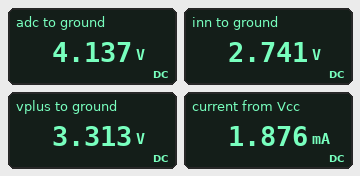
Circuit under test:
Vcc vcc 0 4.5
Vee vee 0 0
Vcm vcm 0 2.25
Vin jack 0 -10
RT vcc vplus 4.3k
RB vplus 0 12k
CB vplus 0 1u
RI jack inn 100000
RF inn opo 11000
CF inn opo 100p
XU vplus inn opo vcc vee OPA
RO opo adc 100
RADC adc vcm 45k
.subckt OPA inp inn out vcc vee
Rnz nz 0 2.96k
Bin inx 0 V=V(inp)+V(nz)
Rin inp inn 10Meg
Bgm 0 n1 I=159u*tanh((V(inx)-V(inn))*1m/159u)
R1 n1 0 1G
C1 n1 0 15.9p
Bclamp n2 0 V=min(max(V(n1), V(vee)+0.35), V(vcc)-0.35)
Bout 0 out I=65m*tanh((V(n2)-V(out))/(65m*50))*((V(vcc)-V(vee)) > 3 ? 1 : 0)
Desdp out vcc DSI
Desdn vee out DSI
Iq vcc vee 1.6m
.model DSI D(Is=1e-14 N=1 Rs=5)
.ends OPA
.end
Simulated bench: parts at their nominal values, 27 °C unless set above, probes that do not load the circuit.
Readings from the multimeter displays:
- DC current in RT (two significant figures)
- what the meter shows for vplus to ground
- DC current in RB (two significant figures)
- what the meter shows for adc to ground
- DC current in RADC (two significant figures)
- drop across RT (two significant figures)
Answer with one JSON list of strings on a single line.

["280 µA", "3.313 V", "280 µA", "4.137 V", "42 µA", "1.2 V"]
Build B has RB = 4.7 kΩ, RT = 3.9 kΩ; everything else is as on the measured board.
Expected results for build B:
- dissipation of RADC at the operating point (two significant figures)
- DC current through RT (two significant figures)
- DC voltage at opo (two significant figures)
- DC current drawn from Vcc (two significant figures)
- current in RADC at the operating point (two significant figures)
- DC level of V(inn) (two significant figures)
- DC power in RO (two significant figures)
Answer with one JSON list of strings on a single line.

["55 µW", "520 µA", "3.8 V", "2.1 mA", "35 µA", "2.5 V", "120 nW"]
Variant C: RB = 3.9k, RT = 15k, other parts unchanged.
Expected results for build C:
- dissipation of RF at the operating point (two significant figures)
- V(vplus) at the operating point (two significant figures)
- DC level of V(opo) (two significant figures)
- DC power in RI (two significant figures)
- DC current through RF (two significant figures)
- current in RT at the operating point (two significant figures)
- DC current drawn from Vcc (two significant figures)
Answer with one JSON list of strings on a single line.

["130 µW", "930 mV", "2.1 V", "1.2 mW", "110 µA", "240 µA", "1.8 mA"]
